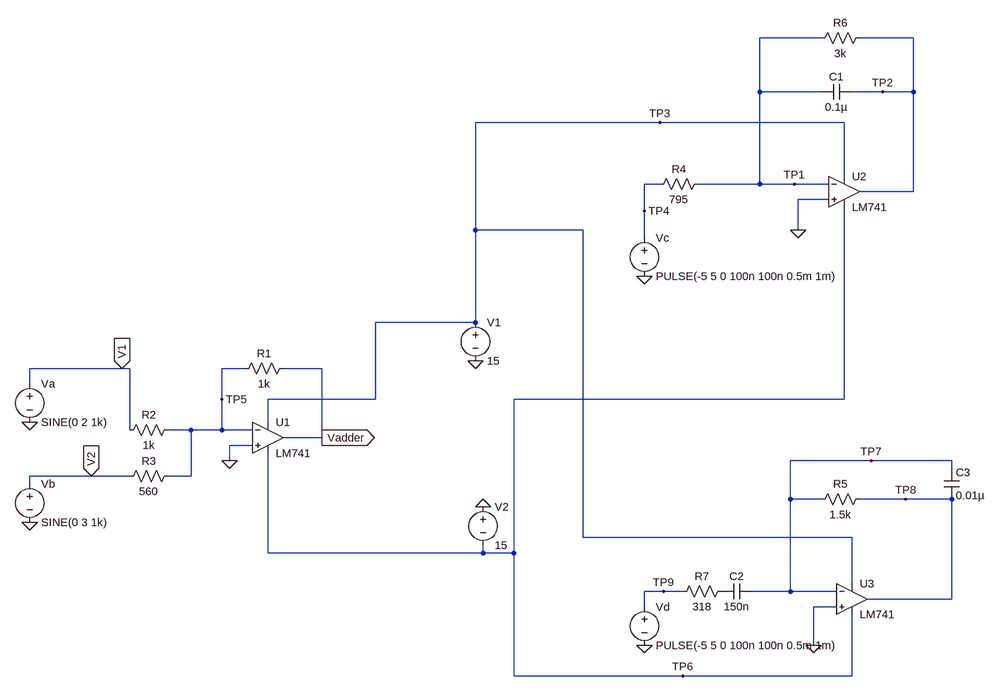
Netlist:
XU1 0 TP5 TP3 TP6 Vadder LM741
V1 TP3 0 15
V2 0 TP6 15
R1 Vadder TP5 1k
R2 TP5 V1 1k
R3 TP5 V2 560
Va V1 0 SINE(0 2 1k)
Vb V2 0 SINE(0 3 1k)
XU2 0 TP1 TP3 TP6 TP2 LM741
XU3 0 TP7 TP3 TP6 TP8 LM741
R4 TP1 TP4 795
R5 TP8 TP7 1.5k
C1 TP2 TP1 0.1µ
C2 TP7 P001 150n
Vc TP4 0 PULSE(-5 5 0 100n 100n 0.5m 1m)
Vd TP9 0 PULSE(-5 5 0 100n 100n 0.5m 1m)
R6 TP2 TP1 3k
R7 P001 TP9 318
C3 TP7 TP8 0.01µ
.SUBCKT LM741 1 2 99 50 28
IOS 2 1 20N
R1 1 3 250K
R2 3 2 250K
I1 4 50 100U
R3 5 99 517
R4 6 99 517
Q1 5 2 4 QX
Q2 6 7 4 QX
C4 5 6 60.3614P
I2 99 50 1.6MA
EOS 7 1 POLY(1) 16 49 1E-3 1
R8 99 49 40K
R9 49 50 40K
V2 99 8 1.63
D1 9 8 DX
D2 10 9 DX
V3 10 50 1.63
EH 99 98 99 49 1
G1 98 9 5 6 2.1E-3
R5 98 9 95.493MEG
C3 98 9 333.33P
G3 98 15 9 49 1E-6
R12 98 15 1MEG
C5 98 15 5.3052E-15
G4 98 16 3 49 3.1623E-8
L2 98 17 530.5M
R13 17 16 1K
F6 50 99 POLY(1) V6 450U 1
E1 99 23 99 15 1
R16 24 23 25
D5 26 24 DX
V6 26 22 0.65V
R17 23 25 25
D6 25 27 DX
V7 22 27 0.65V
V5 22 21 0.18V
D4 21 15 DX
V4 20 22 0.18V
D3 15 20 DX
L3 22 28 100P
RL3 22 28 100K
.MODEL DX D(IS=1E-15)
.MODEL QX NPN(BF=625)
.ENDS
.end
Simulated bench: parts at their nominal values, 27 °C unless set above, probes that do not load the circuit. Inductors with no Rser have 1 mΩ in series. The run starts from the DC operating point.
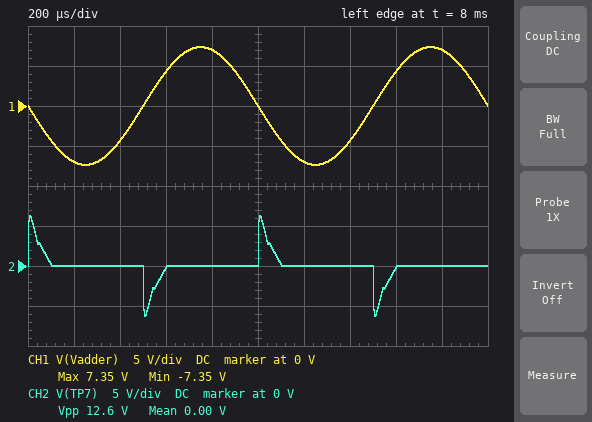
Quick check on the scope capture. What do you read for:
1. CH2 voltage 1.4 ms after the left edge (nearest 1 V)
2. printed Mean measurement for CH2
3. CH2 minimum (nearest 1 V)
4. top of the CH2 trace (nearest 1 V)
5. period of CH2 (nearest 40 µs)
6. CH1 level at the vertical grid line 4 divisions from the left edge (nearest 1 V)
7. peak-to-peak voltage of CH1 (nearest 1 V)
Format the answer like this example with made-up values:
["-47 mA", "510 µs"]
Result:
["0 V", "0.00 V", "-6 V", "6 V", "1.00 ms", "7 V", "15 V"]
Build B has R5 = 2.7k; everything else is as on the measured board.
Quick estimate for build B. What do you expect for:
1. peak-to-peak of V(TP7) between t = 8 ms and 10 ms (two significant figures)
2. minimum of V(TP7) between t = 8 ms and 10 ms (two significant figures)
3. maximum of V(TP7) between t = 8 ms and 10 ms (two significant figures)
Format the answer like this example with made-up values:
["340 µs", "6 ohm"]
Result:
["14 V", "-6.9 V", "6.9 V"]
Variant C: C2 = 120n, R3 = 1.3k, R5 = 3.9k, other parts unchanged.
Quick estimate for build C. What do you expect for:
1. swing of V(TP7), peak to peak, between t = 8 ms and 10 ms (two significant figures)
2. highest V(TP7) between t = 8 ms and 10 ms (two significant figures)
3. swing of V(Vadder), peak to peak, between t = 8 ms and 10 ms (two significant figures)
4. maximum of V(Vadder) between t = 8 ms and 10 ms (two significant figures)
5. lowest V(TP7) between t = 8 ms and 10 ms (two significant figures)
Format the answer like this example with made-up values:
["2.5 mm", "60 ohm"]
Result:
["14 V", "7.1 V", "8.6 V", "4.3 V", "-7.1 V"]
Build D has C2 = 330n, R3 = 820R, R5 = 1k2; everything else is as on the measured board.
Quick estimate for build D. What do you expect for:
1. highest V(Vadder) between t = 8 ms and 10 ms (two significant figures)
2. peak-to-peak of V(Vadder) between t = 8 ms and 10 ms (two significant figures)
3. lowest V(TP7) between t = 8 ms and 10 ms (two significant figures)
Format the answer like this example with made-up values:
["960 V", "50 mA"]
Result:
["5.7 V", "11 V", "-6.3 V"]
